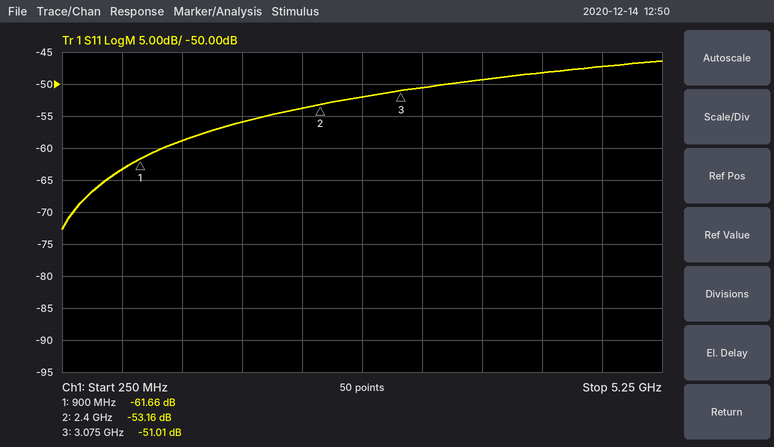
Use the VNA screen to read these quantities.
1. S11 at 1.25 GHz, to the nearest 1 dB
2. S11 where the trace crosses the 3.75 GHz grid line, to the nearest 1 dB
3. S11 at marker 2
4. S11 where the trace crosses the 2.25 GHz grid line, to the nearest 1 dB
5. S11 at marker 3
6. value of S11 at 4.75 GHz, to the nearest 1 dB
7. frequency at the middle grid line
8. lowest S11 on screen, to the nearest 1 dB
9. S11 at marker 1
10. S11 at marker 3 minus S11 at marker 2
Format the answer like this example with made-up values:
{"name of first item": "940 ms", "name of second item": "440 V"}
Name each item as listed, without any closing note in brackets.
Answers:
{"S11 at 1.25 GHz, to the nearest 1 dB": "-59 dB", "S11 where the trace crosses the 3.75 GHz grid line, to the nearest 1 dB": "-49 dB", "S11 at marker 2": "-53.16 dB", "S11 where the trace crosses the 2.25 GHz grid line, to the nearest 1 dB": "-54 dB", "S11 at marker 3": "-51.01 dB", "value of S11 at 4.75 GHz, to the nearest 1 dB": "-47 dB", "frequency at the middle grid line": "2.75 GHz", "lowest S11 on screen, to the nearest 1 dB": "-73 dB", "S11 at marker 1": "-61.66 dB", "S11 at marker 3 minus S11 at marker 2": "2.15 dB"}
